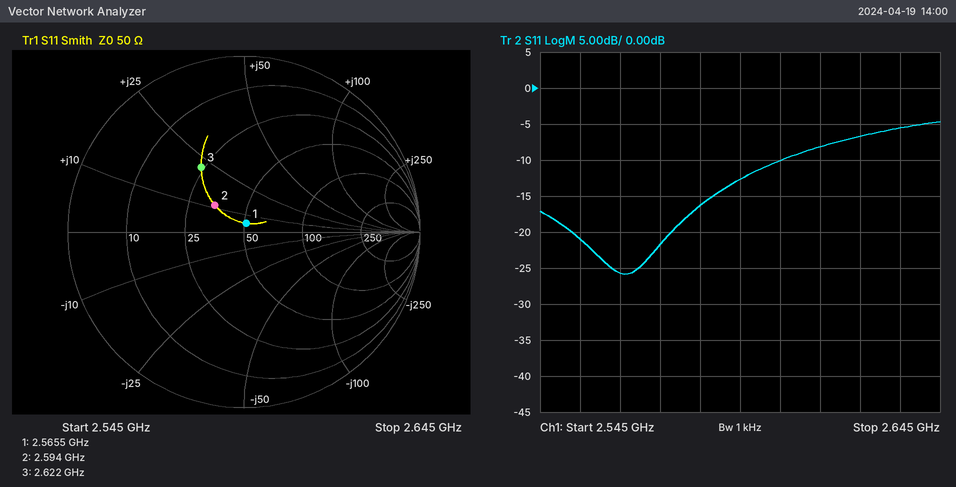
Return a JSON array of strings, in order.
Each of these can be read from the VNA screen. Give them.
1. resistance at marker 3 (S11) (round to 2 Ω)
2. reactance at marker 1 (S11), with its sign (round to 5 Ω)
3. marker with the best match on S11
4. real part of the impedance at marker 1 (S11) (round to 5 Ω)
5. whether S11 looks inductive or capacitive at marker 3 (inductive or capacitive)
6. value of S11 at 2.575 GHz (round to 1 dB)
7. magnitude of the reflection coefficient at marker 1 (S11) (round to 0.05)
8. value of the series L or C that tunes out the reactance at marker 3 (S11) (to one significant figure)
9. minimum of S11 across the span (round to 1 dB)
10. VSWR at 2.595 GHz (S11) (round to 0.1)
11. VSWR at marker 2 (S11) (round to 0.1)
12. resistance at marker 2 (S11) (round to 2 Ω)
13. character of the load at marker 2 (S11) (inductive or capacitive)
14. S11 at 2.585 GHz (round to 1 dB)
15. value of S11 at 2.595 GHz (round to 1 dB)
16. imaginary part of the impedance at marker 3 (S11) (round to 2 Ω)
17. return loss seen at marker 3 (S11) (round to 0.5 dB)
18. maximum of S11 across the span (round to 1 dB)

["24 Ω", "+5 Ω", "marker 1", "50 Ω", "inductive", "-22 dB", "0.05", "3 pF", "-26 dB", "1.6", "1.6", "34 Ω", "inductive", "-16 dB", "-13 dB", "+22 Ω", "7.0 dB", "-5 dB"]
